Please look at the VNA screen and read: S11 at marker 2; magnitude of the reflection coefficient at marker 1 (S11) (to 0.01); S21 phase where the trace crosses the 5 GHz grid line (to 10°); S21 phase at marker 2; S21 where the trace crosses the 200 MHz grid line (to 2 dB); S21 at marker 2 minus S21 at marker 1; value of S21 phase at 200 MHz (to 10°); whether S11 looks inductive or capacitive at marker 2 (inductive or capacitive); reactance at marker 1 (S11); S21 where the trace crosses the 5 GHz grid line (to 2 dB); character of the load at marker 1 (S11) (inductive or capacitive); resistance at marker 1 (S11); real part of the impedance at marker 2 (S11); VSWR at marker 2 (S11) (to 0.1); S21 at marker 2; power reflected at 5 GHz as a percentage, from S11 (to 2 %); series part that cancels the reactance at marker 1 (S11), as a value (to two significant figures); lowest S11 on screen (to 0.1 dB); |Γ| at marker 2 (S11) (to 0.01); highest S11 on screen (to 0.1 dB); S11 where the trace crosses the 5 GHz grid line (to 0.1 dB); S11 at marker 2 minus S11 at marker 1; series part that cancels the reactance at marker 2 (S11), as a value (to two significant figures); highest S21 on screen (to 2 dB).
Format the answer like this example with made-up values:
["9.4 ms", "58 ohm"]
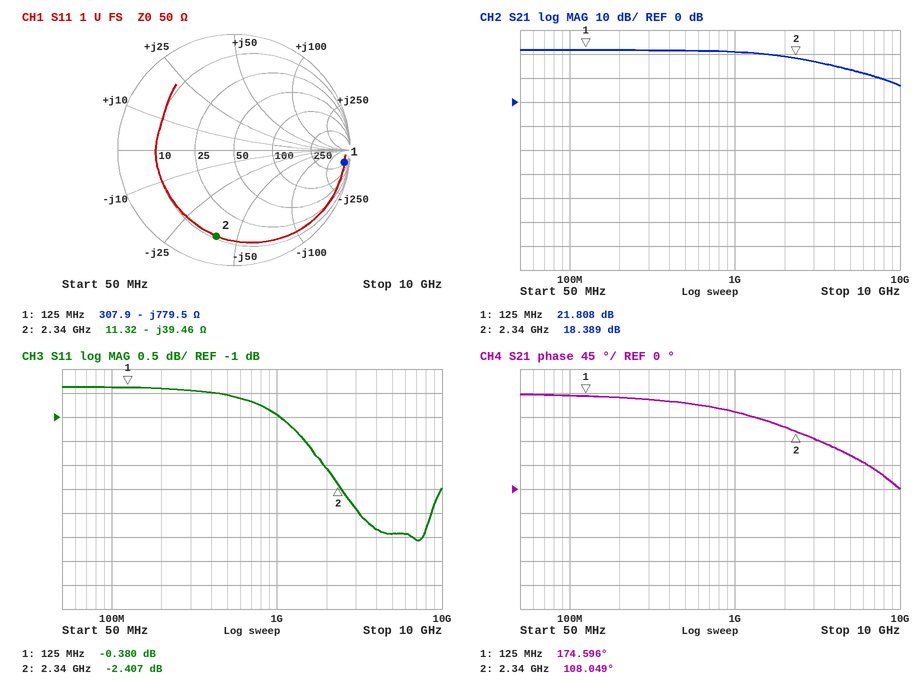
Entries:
["-2.407 dB", "0.96", "60°", "108.049°", "22 dB", "-3.419 dB", "170°", "capacitive", "-779.5 Ω", "14 dB", "capacitive", "307.9 Ω", "11.32 Ω", "7.3", "18.389 dB", "46 %", "990 nH", "-3.6 dB", "0.76", "-0.4 dB", "-3.4 dB", "-2.027 dB", "2.7 nH", "22 dB"]
